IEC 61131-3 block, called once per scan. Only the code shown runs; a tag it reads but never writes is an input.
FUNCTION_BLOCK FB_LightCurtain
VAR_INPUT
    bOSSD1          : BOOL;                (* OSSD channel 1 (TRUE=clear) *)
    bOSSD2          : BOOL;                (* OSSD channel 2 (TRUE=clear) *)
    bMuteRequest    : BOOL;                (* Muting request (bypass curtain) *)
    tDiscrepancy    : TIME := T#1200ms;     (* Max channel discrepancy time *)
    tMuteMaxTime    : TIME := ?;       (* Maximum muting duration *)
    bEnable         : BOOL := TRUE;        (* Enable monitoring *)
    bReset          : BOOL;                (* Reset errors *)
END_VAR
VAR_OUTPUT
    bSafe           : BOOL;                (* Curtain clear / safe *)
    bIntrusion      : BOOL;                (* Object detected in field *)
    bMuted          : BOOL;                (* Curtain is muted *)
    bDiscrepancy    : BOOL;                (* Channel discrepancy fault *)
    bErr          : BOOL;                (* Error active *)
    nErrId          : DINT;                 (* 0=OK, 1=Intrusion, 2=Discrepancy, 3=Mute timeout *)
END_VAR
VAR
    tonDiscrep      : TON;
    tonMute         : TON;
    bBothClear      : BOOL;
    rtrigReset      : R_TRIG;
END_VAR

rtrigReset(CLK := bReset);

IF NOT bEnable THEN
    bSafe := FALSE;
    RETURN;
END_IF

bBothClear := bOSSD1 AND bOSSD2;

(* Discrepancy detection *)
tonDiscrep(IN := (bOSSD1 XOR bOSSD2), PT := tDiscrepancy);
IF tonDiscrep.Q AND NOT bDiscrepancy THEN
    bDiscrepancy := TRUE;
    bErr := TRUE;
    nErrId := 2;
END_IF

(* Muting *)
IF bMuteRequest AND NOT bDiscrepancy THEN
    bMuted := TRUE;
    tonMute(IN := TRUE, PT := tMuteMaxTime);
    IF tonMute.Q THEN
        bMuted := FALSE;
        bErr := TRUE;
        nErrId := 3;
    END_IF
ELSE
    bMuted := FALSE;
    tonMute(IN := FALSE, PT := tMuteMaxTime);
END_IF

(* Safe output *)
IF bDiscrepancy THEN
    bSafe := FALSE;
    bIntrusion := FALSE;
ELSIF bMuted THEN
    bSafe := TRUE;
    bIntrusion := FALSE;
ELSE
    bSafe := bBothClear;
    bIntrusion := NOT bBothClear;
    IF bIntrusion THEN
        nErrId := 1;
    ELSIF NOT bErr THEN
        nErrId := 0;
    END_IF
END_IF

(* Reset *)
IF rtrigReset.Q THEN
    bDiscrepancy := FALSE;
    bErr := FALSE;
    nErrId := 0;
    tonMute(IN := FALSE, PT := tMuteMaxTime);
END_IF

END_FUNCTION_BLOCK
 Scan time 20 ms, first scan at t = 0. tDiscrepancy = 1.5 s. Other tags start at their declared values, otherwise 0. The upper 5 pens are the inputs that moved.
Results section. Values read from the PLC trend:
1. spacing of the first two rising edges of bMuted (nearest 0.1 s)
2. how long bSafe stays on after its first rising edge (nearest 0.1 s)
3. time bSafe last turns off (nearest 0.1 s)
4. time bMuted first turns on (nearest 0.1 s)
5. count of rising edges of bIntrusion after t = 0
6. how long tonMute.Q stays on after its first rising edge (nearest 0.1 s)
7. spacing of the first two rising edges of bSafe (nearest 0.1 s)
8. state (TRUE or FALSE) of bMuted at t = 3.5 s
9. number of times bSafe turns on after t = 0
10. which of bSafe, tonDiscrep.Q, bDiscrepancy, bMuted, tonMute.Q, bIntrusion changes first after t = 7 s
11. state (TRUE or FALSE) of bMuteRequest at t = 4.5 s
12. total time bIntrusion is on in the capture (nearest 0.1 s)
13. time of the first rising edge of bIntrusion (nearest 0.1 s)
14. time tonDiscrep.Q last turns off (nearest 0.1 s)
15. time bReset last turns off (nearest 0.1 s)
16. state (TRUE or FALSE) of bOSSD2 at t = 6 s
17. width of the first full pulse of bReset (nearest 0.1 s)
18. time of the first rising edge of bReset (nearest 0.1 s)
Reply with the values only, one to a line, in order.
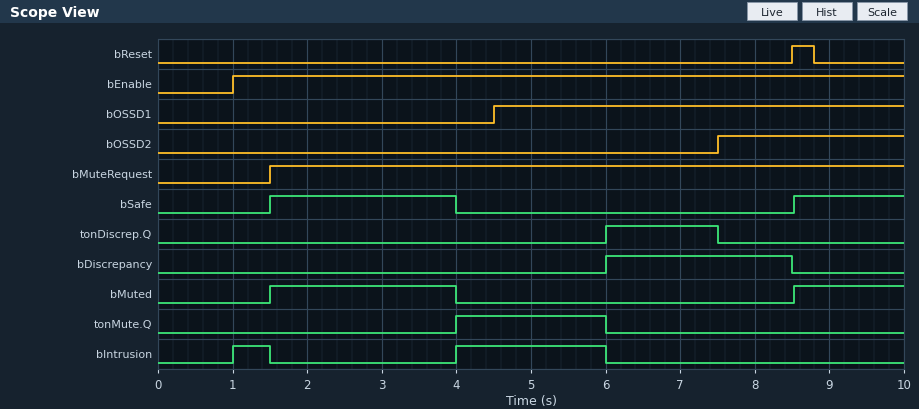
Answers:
7.0 s
2.5 s
4.0 s
1.5 s
2
2.0 s
7.0 s
TRUE
2
tonDiscrep.Q
TRUE
2.5 s
1.0 s
7.5 s
8.8 s
FALSE
0.3 s
8.5 s
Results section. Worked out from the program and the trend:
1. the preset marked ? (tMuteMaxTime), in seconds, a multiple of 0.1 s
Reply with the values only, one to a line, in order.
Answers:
2.5 s
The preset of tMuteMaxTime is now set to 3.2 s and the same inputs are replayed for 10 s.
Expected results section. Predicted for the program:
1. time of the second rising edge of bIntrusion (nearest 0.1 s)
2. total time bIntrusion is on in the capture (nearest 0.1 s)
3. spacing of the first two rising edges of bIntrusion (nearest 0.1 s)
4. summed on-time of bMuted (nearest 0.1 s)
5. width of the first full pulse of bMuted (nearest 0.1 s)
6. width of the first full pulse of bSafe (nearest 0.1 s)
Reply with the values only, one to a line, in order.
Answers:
4.7 s
1.8 s
3.7 s
4.7 s
3.2 s
3.2 s
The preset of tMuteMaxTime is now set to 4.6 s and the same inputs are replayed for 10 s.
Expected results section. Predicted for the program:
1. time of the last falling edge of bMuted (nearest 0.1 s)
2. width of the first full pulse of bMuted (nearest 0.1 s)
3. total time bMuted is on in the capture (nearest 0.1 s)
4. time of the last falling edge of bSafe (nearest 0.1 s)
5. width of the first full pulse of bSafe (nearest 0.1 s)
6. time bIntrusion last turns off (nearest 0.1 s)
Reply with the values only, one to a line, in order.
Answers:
6.0 s
4.5 s
6.0 s
6.0 s
4.5 s
1.5 s
